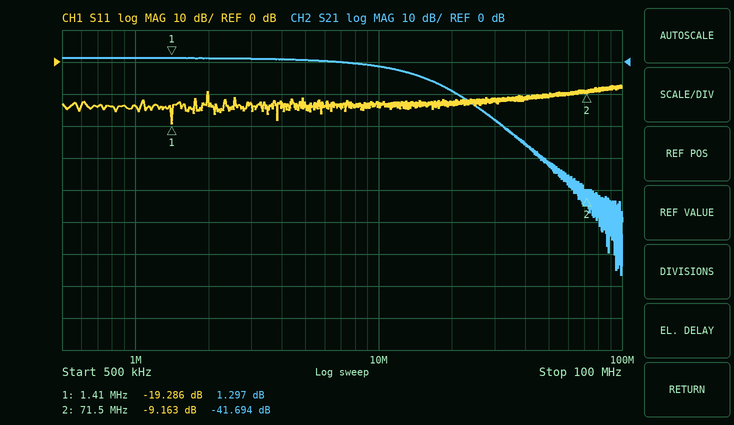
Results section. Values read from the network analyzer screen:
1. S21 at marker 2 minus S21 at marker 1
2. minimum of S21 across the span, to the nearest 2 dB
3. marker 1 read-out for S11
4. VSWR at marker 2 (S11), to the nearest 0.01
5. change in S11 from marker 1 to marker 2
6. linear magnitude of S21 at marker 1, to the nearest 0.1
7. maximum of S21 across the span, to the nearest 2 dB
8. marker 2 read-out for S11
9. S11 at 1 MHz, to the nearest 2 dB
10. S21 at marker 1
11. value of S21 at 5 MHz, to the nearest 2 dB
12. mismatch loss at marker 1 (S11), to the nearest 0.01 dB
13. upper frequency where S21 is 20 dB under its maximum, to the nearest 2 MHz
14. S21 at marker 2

-42.991 dB
-66 dB
-19.286 dB
2.07
10.123 dB
1.2
2 dB
-9.163 dB
-14 dB
1.297 dB
0 dB
0.05 dB
30 MHz
-41.694 dB
